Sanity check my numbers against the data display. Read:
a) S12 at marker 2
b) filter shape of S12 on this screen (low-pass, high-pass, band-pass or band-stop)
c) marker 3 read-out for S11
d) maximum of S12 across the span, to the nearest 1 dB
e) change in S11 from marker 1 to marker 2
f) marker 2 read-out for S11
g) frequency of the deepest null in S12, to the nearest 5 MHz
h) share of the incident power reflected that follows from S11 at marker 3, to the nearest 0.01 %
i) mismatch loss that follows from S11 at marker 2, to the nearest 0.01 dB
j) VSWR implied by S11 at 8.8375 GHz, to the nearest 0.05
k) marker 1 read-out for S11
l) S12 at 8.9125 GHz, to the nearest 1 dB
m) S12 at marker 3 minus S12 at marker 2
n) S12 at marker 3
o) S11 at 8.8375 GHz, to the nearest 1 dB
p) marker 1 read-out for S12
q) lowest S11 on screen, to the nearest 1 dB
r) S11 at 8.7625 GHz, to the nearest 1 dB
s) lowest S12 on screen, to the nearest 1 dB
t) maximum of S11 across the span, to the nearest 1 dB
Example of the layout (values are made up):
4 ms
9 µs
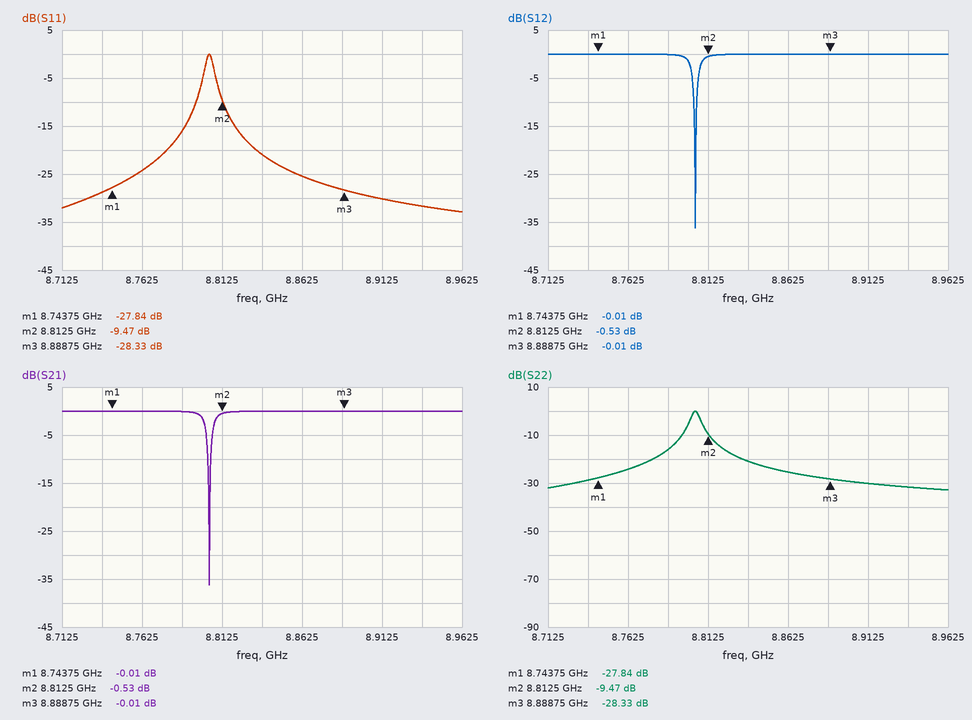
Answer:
-0.53 dB
band-stop
-28.33 dB
0 dB
18.37 dB
-9.47 dB
8.805 GHz
0.15 %
0.52 dB
1.20
-27.84 dB
0 dB
0.52 dB
-0.01 dB
-21 dB
-0.01 dB
-33 dB
-24 dB
-36 dB
0 dB
